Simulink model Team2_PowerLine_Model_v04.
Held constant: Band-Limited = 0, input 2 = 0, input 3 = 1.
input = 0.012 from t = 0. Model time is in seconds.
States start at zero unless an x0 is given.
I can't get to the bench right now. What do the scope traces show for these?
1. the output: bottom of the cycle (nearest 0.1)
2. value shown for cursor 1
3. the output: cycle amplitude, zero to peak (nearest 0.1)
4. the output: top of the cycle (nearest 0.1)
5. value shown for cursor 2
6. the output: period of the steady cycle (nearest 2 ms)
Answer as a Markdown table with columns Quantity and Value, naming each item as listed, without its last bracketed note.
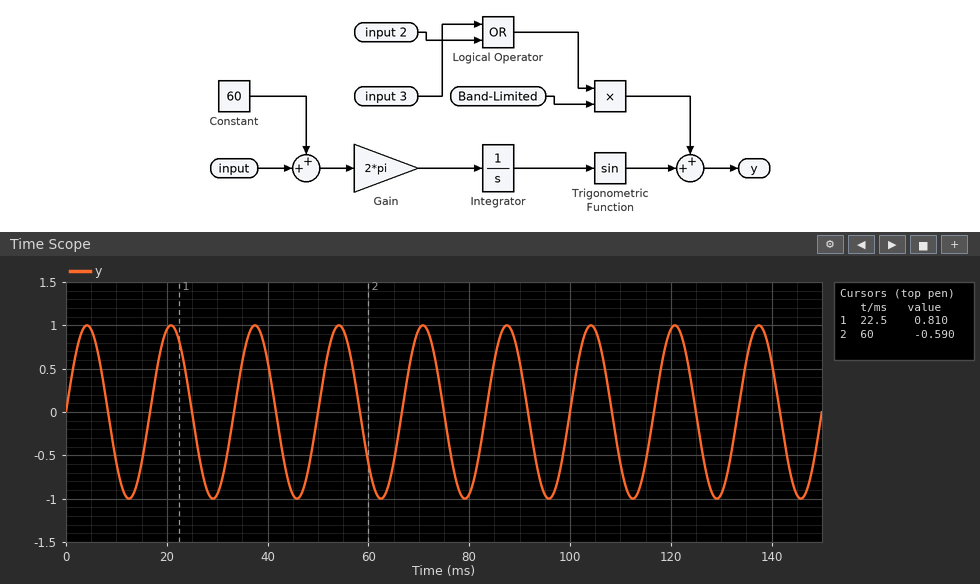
| Quantity | Value |
|---|---|
| the output: bottom of the cycle | -1.0 |
| value shown for cursor 1 | 0.810 |
| the output: cycle amplitude, zero to peak | 1.0 |
| the output: top of the cycle | 1.0 |
| value shown for cursor 2 | -0.590 |
| the output: period of the steady cycle | 16 ms |
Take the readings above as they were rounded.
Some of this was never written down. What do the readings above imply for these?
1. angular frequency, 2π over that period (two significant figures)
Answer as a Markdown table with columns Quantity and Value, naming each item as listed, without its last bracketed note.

| Quantity | Value |
|---|---|
| angular frequency, 2π over that period | 0.39 rad/ms |
